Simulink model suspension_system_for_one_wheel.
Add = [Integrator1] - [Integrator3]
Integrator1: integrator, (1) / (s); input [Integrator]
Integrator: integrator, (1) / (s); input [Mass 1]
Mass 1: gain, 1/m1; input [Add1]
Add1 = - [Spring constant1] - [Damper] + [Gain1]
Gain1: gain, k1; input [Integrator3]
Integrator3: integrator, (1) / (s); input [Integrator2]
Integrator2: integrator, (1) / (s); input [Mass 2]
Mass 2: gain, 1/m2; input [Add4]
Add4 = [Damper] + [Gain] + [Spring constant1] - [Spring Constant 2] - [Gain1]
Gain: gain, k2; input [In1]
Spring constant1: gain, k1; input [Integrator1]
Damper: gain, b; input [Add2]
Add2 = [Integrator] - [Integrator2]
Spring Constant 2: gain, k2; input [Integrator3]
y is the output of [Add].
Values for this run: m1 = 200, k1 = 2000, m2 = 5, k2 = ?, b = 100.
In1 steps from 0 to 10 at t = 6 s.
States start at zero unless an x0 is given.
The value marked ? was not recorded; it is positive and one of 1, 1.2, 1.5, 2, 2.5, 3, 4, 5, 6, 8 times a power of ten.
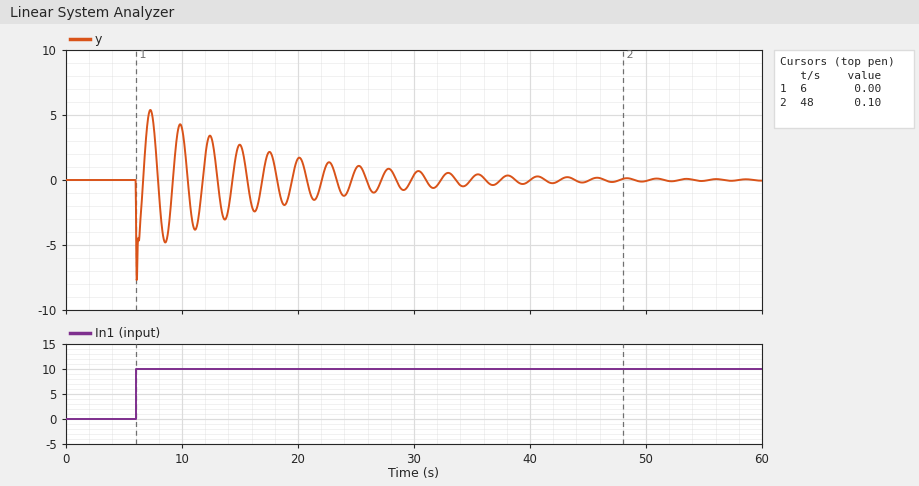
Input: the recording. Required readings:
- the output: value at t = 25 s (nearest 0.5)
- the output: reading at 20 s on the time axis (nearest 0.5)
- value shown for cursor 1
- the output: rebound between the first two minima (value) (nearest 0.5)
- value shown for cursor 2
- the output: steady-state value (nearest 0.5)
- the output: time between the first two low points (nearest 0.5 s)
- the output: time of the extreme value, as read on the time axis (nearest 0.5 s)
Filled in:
1.0
1.5
0.00
5.5
0.10
0.0
2.5 s
6.0 s
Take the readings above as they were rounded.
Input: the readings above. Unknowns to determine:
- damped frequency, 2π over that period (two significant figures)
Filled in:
2.5 rad/s
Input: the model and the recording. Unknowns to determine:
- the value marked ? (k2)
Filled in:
3000
